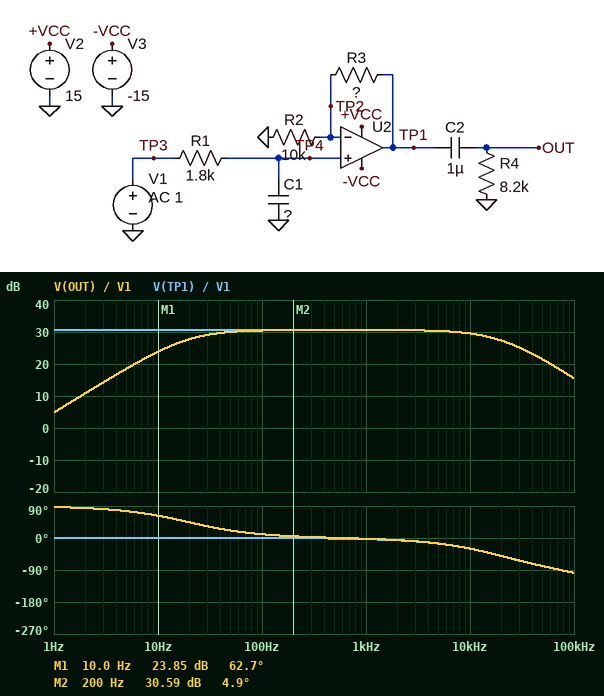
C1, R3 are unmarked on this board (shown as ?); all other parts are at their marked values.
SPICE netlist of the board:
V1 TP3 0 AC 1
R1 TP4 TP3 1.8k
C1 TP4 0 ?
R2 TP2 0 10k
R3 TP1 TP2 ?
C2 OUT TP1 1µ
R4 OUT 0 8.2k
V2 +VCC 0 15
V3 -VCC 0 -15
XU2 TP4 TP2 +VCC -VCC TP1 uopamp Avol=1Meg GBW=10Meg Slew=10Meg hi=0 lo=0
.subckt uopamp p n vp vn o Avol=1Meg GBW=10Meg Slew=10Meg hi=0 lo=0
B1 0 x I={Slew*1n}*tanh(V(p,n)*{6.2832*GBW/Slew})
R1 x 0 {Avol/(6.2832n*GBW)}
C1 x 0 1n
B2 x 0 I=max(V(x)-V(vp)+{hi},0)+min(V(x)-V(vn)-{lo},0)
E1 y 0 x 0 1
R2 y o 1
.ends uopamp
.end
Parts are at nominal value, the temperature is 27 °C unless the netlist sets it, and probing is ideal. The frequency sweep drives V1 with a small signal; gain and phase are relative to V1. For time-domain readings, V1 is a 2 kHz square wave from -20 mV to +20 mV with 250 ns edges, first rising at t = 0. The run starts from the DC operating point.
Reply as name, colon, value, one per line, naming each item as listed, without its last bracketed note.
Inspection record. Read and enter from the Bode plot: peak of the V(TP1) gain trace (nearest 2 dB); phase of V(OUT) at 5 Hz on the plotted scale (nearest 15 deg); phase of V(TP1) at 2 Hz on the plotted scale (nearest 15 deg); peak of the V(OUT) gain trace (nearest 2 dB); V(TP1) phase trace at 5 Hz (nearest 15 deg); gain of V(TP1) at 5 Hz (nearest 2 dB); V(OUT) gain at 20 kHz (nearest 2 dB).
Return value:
peak of the V(TP1) gain trace: 30 dB
phase of V(OUT) at 5 Hz on the plotted scale: 75 deg
phase of V(TP1) at 2 Hz on the plotted scale: 0 deg
peak of the V(OUT) gain trace: 30 dB
V(TP1) phase trace at 5 Hz: 0 deg
gain of V(TP1) at 5 Hz: 30 dB
V(OUT) gain at 20 kHz: 28 dB
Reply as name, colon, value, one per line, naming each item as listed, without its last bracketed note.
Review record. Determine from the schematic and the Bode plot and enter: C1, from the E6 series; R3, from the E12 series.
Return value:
C1, from the E6 series: 4.7 nF
R3, from the E12 series: 330 kΩ
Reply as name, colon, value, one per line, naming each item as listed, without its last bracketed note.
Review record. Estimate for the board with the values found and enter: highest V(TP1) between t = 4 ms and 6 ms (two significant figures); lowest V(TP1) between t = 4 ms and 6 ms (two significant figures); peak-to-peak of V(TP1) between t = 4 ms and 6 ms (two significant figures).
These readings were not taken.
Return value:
highest V(TP1) between t = 4 ms and 6 ms: 680 mV
lowest V(TP1) between t = 4 ms and 6 ms: -680 mV
peak-to-peak of V(TP1) between t = 4 ms and 6 ms: 1.4 V
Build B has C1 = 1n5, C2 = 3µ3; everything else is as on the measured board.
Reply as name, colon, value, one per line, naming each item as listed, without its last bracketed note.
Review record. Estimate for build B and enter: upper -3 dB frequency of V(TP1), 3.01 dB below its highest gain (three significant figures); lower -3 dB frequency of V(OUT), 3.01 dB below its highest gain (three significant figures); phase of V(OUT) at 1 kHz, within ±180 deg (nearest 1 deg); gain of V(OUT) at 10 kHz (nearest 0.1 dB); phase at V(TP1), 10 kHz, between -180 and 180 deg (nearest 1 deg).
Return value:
upper -3 dB frequency of V(TP1), 3.01 dB below its highest gain: 56.8 kHz
lower -3 dB frequency of V(OUT), 3.01 dB below its highest gain: 5.88 Hz
phase of V(OUT) at 1 kHz, within ±180 deg: -1 deg
gain of V(OUT) at 10 kHz: 30.5 dB
phase at V(TP1), 10 kHz, between -180 and 180 deg: -12 deg
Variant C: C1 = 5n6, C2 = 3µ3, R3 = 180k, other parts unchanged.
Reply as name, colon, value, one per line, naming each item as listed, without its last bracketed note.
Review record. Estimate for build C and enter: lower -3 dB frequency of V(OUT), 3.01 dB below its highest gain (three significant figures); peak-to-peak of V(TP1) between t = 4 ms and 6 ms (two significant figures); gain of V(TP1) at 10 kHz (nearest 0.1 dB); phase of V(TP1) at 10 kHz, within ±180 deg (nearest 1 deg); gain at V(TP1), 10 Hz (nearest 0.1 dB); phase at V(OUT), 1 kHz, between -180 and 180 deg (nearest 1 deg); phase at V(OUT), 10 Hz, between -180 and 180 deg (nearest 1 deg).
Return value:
lower -3 dB frequency of V(OUT), 3.01 dB below its highest gain: 5.88 Hz
peak-to-peak of V(TP1) between t = 4 ms and 6 ms: 760 mV
gain of V(TP1) at 10 kHz: 24.1 dB
phase of V(TP1) at 10 kHz, within ±180 deg: -33 deg
gain at V(TP1), 10 Hz: 25.6 dB
phase at V(OUT), 1 kHz, between -180 and 180 deg: -3 deg
phase at V(OUT), 10 Hz, between -180 and 180 deg: 30 deg
